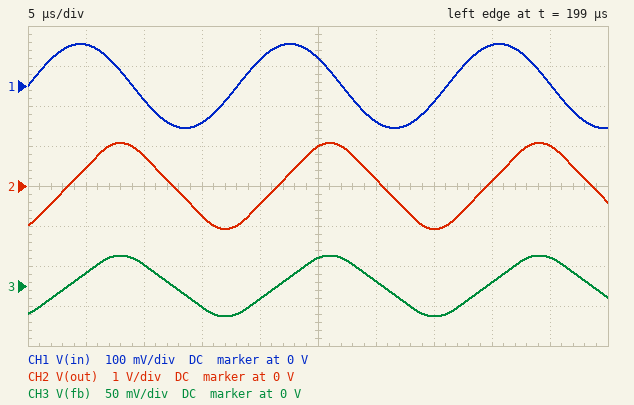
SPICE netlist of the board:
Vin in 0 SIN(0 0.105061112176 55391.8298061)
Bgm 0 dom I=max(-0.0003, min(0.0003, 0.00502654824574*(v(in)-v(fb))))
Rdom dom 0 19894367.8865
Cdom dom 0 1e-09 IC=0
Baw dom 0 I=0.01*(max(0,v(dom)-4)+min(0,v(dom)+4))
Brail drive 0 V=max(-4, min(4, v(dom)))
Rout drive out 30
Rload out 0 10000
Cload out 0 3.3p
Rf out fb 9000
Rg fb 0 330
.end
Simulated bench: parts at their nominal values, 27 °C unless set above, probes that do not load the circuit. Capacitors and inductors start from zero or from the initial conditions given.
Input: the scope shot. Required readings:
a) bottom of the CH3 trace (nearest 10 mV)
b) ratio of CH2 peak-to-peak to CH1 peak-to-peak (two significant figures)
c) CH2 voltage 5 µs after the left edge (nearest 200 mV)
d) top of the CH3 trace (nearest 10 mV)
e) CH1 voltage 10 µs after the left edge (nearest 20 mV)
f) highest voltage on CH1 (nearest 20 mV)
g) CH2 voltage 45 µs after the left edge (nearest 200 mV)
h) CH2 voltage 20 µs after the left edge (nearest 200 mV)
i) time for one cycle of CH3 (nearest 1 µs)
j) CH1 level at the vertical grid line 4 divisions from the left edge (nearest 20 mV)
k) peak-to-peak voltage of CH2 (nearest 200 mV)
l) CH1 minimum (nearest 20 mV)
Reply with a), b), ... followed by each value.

a) -40 mV
b) 10
c) 400 mV
d) 40 mV
e) -40 mV
f) 100 mV
g) 1.0 V
h) -400 mV
i) 18 µs
j) 60 mV
k) 2.2 V
l) -100 mV
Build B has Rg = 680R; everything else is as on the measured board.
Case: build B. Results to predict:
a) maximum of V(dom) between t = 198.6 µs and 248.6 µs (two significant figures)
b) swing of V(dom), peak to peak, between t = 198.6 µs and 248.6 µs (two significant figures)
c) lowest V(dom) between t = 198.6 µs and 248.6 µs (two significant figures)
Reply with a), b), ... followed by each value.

a) 1.0 V
b) 2.0 V
c) -1.0 V
